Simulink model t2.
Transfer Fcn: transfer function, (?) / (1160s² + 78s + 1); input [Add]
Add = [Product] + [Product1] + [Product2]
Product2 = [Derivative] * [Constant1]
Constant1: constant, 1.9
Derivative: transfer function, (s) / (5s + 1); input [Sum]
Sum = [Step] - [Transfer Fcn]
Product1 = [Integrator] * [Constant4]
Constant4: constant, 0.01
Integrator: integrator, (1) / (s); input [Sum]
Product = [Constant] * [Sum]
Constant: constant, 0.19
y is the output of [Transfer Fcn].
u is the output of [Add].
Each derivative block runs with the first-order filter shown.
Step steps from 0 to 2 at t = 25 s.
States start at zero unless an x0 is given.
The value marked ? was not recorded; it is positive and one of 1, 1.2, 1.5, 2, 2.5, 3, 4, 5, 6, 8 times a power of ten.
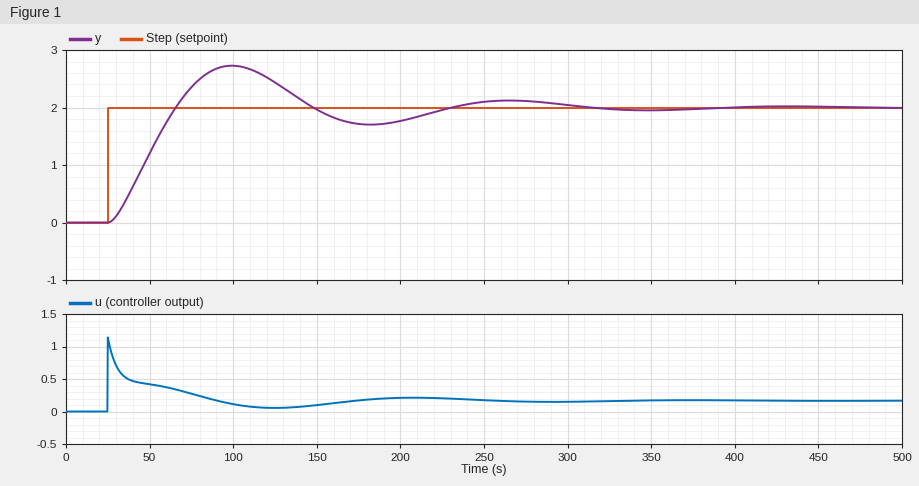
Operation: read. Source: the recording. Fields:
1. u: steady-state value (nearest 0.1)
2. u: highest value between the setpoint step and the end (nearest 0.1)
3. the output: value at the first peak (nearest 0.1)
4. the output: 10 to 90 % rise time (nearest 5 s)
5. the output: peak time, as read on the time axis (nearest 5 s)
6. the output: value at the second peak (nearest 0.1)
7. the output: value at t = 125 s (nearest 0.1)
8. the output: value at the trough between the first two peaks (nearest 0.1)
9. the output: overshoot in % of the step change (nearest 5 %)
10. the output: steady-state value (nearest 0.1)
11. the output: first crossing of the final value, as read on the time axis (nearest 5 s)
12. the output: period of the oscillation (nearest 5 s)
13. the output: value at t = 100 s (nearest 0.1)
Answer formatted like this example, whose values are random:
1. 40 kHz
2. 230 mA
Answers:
1. 0.2
2. 1.1
3. 2.7
4. 30 s
5. 100 s
6. 2.1
7. 2.4
8. 1.7
9. 35 %
10. 2.0
11. 65 s
12. 165 s
13. 2.7
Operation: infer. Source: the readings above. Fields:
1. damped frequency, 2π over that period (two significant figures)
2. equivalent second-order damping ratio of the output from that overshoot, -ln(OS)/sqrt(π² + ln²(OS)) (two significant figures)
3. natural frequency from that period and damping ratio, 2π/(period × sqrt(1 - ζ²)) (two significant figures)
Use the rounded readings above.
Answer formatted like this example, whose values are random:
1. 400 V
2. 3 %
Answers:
1. 0.038 rad/s
2. 0.32
3. 0.040 rad/s
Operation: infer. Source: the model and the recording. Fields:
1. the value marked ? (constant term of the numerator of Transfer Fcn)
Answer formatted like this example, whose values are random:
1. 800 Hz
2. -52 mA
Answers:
1. 12
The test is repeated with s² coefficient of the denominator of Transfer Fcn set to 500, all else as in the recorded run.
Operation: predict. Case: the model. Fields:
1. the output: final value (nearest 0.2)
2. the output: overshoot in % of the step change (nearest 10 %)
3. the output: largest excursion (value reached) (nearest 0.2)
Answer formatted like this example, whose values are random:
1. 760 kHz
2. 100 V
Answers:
1. 2.0
2. 20 %
3. 2.4
